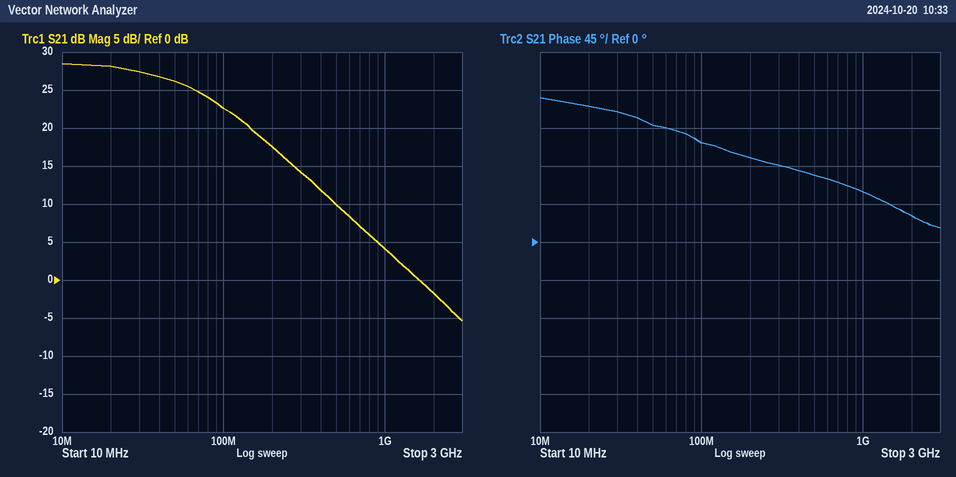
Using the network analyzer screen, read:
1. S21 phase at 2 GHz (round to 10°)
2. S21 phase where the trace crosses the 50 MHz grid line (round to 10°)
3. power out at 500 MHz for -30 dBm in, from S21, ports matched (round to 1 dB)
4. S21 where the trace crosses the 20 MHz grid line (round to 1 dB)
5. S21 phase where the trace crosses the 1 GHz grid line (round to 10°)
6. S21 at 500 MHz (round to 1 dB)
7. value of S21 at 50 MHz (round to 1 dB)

30°
140°
-20 dBm
28 dB
60°
10 dB
26 dB
